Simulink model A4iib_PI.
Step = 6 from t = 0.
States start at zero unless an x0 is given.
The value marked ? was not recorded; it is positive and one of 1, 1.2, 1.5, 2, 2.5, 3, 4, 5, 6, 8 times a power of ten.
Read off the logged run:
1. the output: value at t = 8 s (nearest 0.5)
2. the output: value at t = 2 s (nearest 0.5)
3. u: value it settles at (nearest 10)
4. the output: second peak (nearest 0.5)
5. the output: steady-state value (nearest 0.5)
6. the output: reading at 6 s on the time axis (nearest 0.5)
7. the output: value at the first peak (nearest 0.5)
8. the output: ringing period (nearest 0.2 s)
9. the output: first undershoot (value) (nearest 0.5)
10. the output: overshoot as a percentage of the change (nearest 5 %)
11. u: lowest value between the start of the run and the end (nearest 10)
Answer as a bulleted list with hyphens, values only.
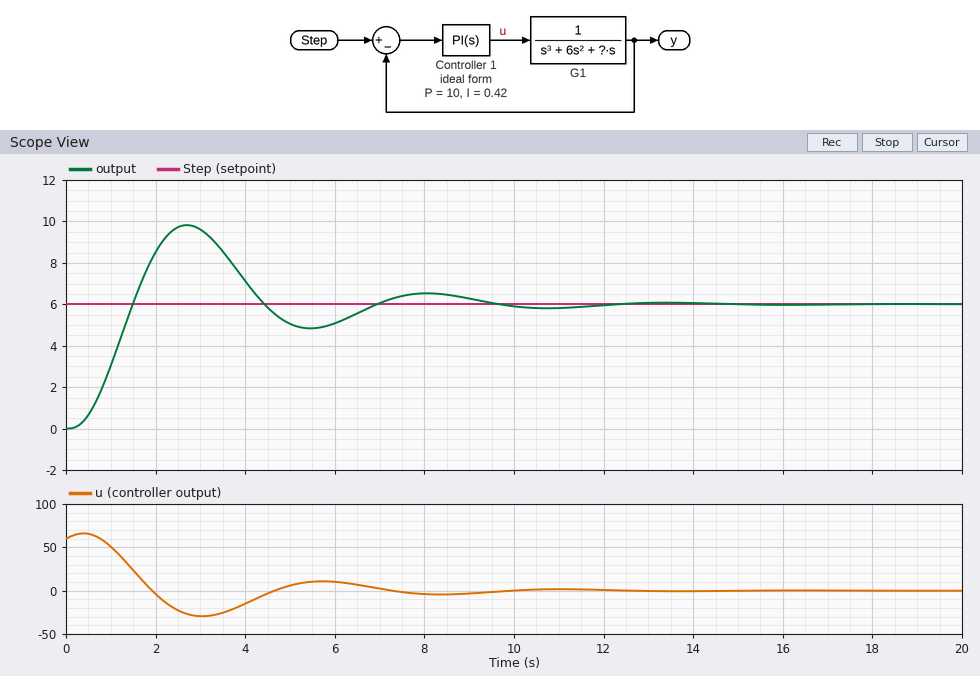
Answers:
- 6.5
- 8.5
- 0
- 6.5
- 6.0
- 5.0
- 10.0
- 5.4 s
- 5.0
- 65 %
- -30
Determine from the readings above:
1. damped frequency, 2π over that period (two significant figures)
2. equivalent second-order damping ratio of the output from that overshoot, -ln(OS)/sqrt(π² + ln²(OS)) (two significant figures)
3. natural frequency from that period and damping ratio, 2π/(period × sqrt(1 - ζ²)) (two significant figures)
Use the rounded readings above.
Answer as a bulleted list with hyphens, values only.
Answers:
- 1.2 rad/s
- 0.14
- 1.2 rad/s
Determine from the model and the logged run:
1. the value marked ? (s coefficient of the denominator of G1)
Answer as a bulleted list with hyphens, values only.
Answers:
- 8
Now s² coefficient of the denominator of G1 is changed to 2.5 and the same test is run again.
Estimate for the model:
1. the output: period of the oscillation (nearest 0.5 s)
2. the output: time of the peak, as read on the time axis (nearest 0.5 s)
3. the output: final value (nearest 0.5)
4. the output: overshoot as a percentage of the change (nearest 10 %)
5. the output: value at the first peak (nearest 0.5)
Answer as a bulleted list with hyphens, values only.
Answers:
- 2.5 s
- 2.0 s
- 6.0
- 50 %
- 9.0
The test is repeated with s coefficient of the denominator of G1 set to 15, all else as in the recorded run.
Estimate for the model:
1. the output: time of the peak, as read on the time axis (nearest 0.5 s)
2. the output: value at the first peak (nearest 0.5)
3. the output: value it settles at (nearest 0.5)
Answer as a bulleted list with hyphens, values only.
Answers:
- 4.0 s
- 8.0
- 6.0
